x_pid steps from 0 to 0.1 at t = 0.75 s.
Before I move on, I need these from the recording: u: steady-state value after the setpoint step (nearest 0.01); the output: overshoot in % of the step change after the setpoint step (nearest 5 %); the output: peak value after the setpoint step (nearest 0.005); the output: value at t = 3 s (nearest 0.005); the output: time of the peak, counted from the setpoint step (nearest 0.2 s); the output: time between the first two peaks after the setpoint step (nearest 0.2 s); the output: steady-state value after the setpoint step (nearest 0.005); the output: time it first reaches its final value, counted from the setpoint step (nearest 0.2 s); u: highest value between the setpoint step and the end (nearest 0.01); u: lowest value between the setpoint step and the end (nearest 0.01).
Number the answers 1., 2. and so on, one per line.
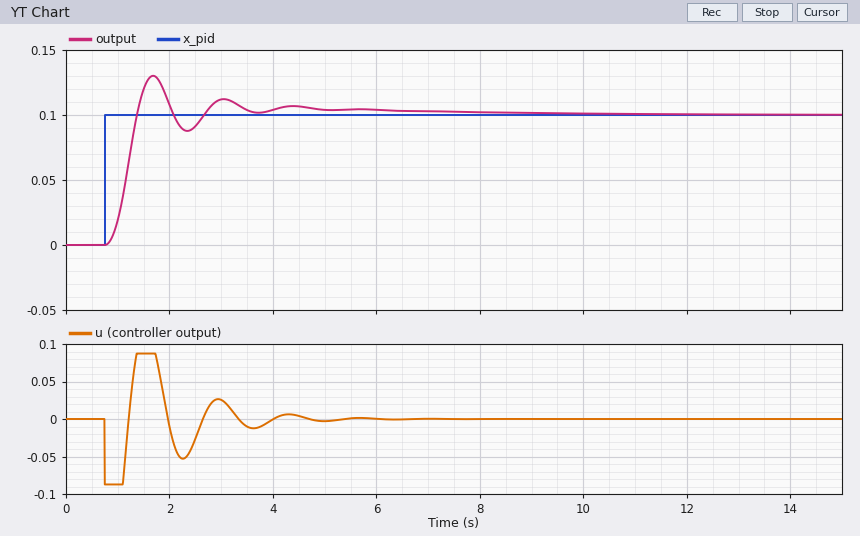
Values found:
1. 0.00
2. 30 %
3. 0.130
4. 0.110
5. 1.0 s
6. 1.4 s
7. 0.100
8. 0.6 s
9. 0.09
10. -0.09
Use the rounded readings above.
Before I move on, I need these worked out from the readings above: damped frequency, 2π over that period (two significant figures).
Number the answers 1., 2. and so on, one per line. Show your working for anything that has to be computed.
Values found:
1. 2π / 1.4 = 4.5 rad/s
